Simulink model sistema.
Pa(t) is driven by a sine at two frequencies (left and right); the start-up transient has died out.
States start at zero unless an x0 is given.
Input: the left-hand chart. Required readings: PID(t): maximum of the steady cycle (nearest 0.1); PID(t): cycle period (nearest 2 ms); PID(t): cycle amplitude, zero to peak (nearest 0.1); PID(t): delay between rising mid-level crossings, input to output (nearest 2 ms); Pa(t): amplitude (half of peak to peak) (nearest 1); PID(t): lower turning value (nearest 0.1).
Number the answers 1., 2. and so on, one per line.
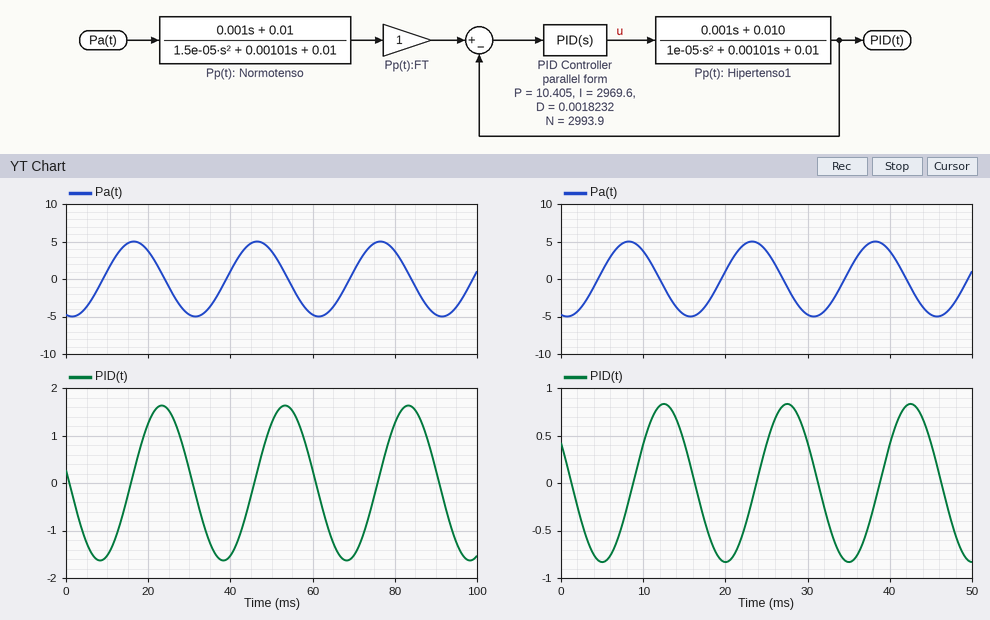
1. 1.6
2. 30 ms
3. 1.6
4. 6 ms
5. 5
6. -1.6
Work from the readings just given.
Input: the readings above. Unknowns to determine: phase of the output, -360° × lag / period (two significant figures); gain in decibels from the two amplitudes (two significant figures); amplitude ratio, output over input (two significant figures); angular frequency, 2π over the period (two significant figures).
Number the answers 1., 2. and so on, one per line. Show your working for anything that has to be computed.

1. -360 × 6 / 30 = -72°
2. 20 log10(1.6 / 5) = -9.9 dB
3. 1.6 / 5 = 0.32
4. 2π / 30 = 0.21 rad/ms
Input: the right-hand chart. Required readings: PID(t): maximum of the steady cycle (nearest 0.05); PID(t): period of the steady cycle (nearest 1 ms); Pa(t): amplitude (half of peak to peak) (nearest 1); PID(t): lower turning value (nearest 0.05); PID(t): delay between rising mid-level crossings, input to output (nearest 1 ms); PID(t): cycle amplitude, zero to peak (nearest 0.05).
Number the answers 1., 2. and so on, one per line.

1. 0.85
2. 15 ms
3. 5
4. -0.85
5. 4 ms
6. 0.85
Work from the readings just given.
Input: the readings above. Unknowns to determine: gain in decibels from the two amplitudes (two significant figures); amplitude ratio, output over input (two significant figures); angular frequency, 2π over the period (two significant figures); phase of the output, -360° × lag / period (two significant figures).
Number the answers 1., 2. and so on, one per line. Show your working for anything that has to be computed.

1. 20 log10(0.85 / 5) = -15 dB
2. 0.85 / 5 = 0.17
3. 2π / 15 = 0.42 rad/ms
4. -360 × 4 / 15 = -96°
